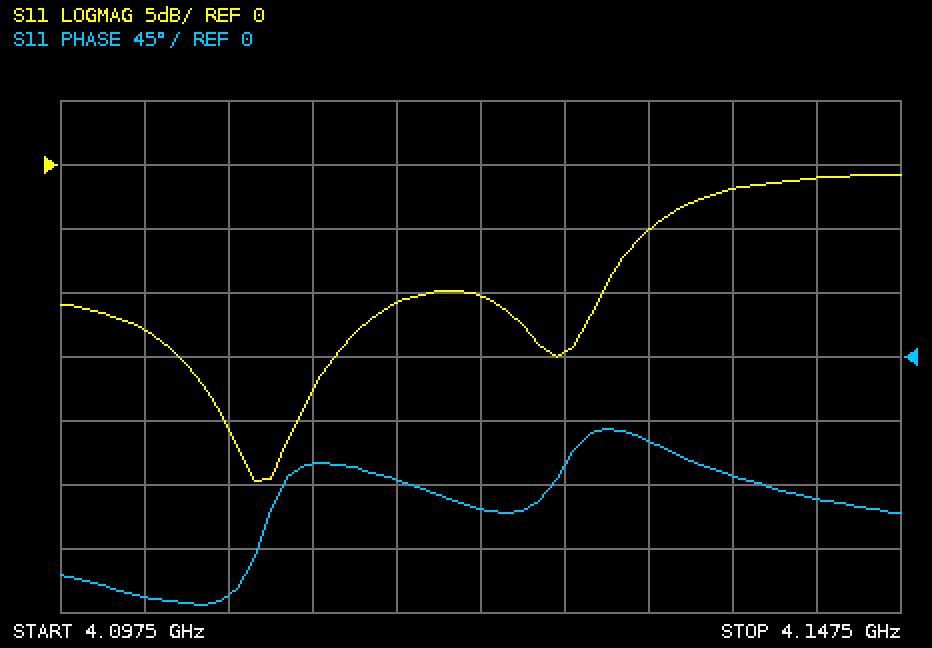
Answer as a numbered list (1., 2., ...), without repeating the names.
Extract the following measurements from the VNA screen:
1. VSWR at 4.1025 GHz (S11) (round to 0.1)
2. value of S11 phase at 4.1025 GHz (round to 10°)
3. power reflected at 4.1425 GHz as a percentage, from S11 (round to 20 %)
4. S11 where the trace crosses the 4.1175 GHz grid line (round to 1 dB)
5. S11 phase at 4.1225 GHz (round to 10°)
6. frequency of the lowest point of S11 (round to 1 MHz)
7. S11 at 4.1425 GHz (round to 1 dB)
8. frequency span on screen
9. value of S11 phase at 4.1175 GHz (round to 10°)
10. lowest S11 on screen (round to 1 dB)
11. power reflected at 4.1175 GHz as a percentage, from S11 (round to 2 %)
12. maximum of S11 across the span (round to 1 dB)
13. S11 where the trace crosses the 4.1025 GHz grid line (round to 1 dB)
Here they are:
1. 1.6
2. -170°
3. 80 %
4. -11 dB
5. -110°
6. 4.109 GHz
7. -1 dB
8. 50 MHz
9. -90°
10. -25 dB
11. 8 %
12. -1 dB
13. -13 dB
